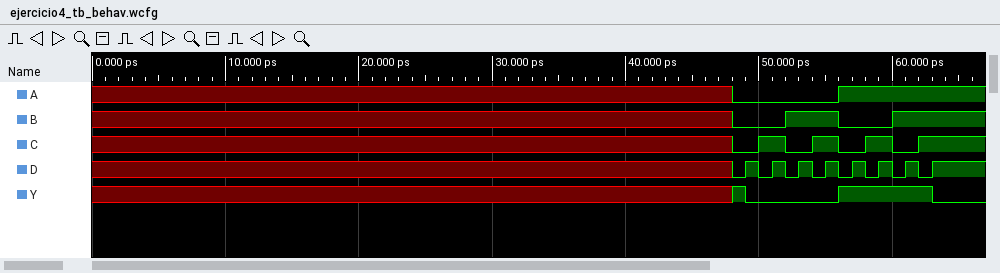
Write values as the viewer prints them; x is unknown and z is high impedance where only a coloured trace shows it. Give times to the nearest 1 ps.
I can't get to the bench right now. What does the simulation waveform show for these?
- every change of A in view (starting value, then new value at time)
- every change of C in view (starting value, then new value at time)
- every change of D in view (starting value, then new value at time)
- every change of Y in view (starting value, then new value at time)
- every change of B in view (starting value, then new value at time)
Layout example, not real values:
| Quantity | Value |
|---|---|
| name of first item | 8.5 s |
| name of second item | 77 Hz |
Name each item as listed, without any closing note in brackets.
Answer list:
| Quantity | Value |
|---|---|
| every change of A in view | x, 0 at 48 ps, 1 at 56 ps |
| every change of C in view | x, 0 at 48 ps, 1 at 50 ps, 0 at 52 ps, 1 at 54 ps, 0 at 56 ps, 1 at 58 ps, 0 at 60 ps, 1 at 62 ps |
| every change of D in view | x, 0 at 48 ps, 1 at 49 ps, 0 at 50 ps, 1 at 51 ps, 0 at 52 ps, 1 at 53 ps, 0 at 54 ps, 1 at 55 ps, 0 at 56 ps, 1 at 57 ps, 0 at 58 ps, 1 at 59 ps, 0 at 60 ps, 1 at 61 ps, 0 at 62 ps, 1 at 63 ps |
| every change of Y in view | x, 1 at 48 ps, 0 at 49 ps, 1 at 56 ps, 0 at 63 ps |
| every change of B in view | x, 0 at 48 ps, 1 at 52 ps, 0 at 56 ps, 1 at 60 ps |
